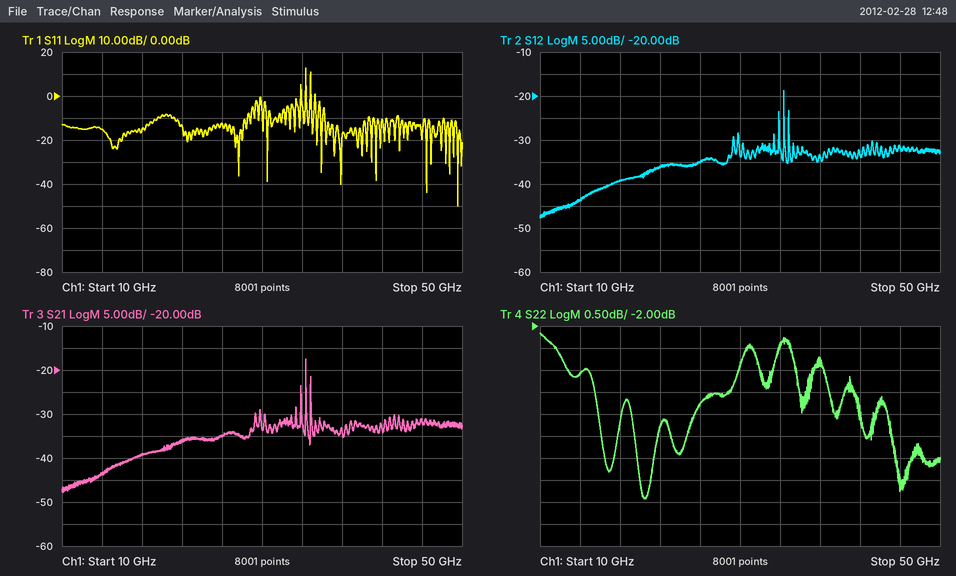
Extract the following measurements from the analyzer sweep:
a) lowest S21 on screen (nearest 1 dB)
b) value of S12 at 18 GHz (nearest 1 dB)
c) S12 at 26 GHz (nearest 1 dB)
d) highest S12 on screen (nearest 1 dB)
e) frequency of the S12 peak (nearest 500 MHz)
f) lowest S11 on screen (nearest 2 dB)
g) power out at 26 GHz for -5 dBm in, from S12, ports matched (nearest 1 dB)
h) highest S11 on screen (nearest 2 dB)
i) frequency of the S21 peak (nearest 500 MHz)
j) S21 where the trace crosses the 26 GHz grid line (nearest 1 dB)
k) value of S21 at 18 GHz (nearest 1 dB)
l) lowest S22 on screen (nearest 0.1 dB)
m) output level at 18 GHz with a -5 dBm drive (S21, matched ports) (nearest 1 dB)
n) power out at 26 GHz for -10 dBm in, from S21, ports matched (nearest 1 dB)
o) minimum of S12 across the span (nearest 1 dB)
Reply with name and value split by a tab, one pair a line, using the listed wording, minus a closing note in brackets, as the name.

lowest S21 on screen	-48 dB
value of S12 at 18 GHz	-39 dB
S12 at 26 GHz	-35 dB
highest S12 on screen	-19 dB
frequency of the S12 peak	34.5 GHz
lowest S11 on screen	-50 dB
power out at 26 GHz for -5 dBm in, from S12, ports matched	-40 dBm
highest S11 on screen	12 dB
frequency of the S21 peak	34.5 GHz
S21 where the trace crosses the 26 GHz grid line	-35 dB
value of S21 at 18 GHz	-39 dB
lowest S22 on screen	-5.9 dB
output level at 18 GHz with a -5 dBm drive (S21, matched ports)	-44 dBm
power out at 26 GHz for -10 dBm in, from S21, ports matched	-45 dBm
minimum of S12 across the span	-48 dB
